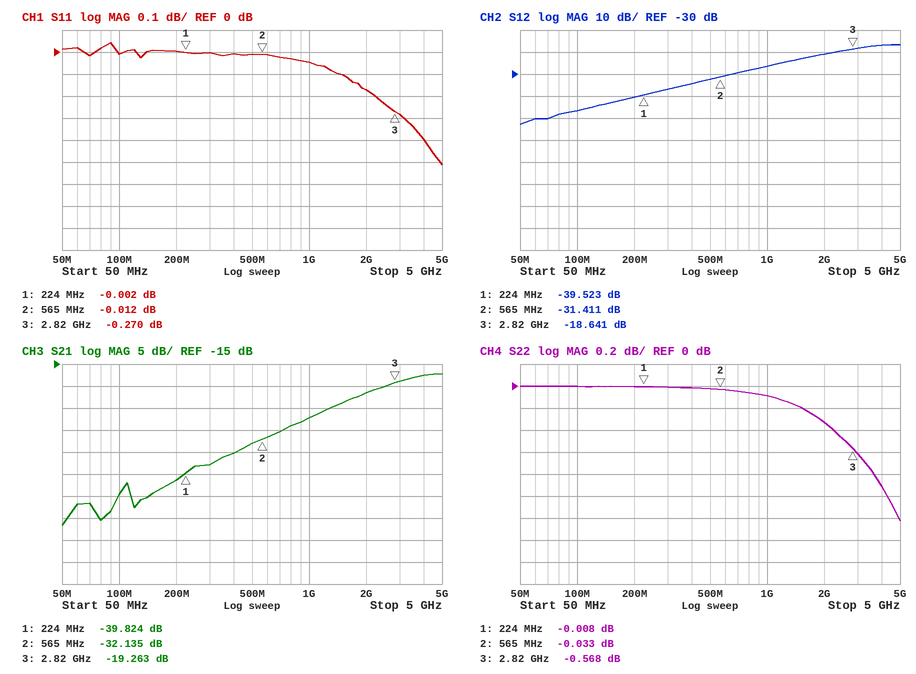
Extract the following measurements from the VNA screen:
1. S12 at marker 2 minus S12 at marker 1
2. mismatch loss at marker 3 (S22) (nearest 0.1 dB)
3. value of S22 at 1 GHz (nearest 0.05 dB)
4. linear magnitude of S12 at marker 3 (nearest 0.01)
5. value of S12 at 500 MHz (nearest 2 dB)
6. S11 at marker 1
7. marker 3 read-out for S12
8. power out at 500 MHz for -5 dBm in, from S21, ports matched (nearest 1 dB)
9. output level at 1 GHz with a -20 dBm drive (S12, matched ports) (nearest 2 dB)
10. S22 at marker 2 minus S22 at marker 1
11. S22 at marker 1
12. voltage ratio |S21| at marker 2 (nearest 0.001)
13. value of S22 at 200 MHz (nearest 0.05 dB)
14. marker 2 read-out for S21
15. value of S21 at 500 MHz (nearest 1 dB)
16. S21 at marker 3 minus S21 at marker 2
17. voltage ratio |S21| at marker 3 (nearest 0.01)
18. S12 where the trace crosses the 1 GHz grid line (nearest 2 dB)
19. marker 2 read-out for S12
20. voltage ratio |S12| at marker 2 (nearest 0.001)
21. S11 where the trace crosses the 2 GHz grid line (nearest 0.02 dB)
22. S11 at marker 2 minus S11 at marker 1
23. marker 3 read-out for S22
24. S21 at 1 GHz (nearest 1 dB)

8.112 dB
9.1 dB
-0.10 dB
0.12
-32 dB
-0.002 dB
-18.641 dB
-38 dBm
-46 dBm
-0.025 dB
-0.008 dB
0.025
0.00 dB
-32.135 dB
-33 dB
12.872 dB
0.11
-26 dB
-31.411 dB
0.027
-0.18 dB
-0.010 dB
-0.568 dB
-27 dB
